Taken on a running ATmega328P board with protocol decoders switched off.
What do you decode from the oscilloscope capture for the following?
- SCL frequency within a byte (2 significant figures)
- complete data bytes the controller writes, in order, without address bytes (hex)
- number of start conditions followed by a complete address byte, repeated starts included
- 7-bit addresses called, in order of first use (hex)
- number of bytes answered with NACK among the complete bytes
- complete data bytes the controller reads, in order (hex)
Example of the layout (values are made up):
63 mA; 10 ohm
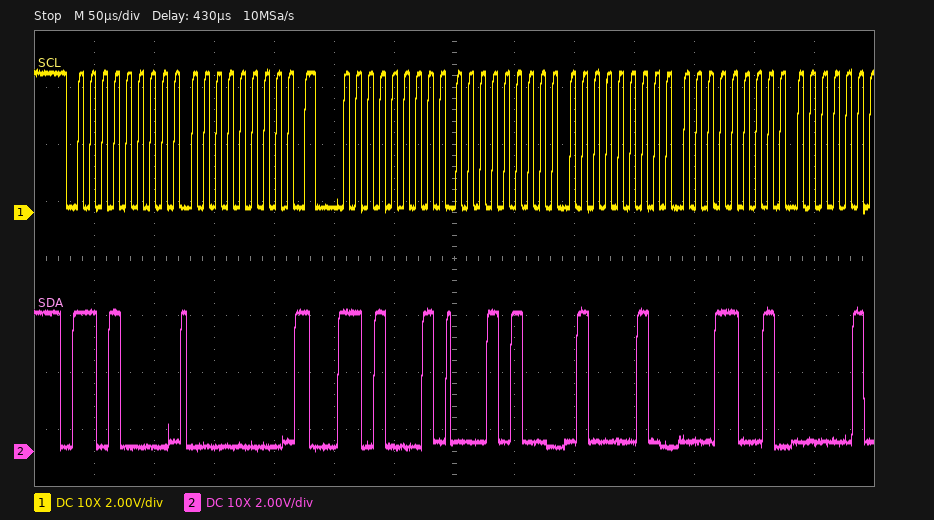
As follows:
100 kHz; 00; 2; 0x68; 0; 14 42 19
